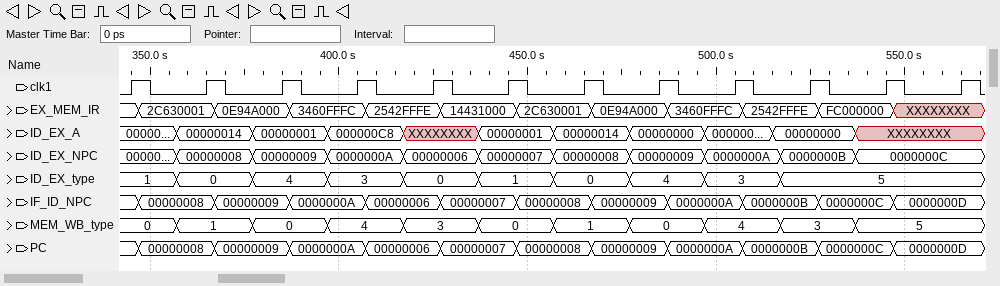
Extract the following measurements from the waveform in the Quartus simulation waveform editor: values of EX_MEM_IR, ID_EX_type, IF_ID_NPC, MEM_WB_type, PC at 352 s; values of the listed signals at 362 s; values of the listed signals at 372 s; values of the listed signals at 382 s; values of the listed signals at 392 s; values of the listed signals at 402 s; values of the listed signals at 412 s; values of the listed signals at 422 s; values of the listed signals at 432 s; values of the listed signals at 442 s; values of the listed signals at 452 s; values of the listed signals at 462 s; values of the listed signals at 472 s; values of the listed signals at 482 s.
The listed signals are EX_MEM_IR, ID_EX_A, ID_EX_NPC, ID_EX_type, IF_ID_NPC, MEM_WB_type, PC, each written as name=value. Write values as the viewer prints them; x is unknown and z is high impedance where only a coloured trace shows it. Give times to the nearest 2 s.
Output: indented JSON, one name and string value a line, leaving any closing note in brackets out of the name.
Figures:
{
  "values of EX_MEM_IR, ID_EX_type, IF_ID_NPC, MEM_WB_type, PC at 352 s": "EX_MEM_IR=2C630001, ID_EX_type=1, IF_ID_NPC=00000008, MEM_WB_type=0, PC=00000008",
  "values of the listed signals at 362 s": "EX_MEM_IR=2C630001, ID_EX_A=00000014, ID_EX_NPC=00000008, ID_EX_type=0, IF_ID_NPC=00000008, MEM_WB_type=1, PC=00000008",
  "values of the listed signals at 372 s": "EX_MEM_IR=0E94A000, ID_EX_A=00000014, ID_EX_NPC=00000008, ID_EX_type=0, IF_ID_NPC=00000009, MEM_WB_type=1, PC=00000009",
  "values of the listed signals at 382 s": "EX_MEM_IR=0E94A000, ID_EX_A=00000001, ID_EX_NPC=00000009, ID_EX_type=4, IF_ID_NPC=00000009, MEM_WB_type=0, PC=00000009",
  "values of the listed signals at 392 s": "EX_MEM_IR=3460FFFC, ID_EX_A=00000001, ID_EX_NPC=00000009, ID_EX_type=4, IF_ID_NPC=0000000A, MEM_WB_type=0, PC=0000000A",
  "values of the listed signals at 402 s": "EX_MEM_IR=3460FFFC, ID_EX_A=000000C8, ID_EX_NPC=0000000A, ID_EX_type=3, IF_ID_NPC=0000000A, MEM_WB_type=4, PC=0000000A",
  "values of the listed signals at 412 s": "EX_MEM_IR=2542FFFE, ID_EX_A=000000C8, ID_EX_NPC=0000000A, ID_EX_type=3, IF_ID_NPC=00000006, MEM_WB_type=4, PC=00000006",
  "values of the listed signals at 422 s": "EX_MEM_IR=2542FFFE, ID_EX_A=XXXXXXXX, ID_EX_NPC=00000006, ID_EX_type=0, IF_ID_NPC=00000006, MEM_WB_type=3, PC=00000006",
  "values of the listed signals at 432 s": "EX_MEM_IR=14431000, ID_EX_A=XXXXXXXX, ID_EX_NPC=00000006, ID_EX_type=0, IF_ID_NPC=00000007, MEM_WB_type=3, PC=00000007",
  "values of the listed signals at 442 s": "EX_MEM_IR=14431000, ID_EX_A=00000001, ID_EX_NPC=00000007, ID_EX_type=1, IF_ID_NPC=00000007, MEM_WB_type=0, PC=00000007",
  "values of the listed signals at 452 s": "EX_MEM_IR=2C630001, ID_EX_A=00000001, ID_EX_NPC=00000007, ID_EX_type=1, IF_ID_NPC=00000008, MEM_WB_type=0, PC=00000008",
  "values of the listed signals at 462 s": "EX_MEM_IR=2C630001, ID_EX_A=00000014, ID_EX_NPC=00000008, ID_EX_type=0, IF_ID_NPC=00000008, MEM_WB_type=1, PC=00000008",
  "values of the listed signals at 472 s": "EX_MEM_IR=0E94A000, ID_EX_A=00000014, ID_EX_NPC=00000008, ID_EX_type=0, IF_ID_NPC=00000009, MEM_WB_type=1, PC=00000009",
  "values of the listed signals at 482 s": "EX_MEM_IR=0E94A000, ID_EX_A=00000000, ID_EX_NPC=00000009, ID_EX_type=4, IF_ID_NPC=00000009, MEM_WB_type=0, PC=00000009"
}
